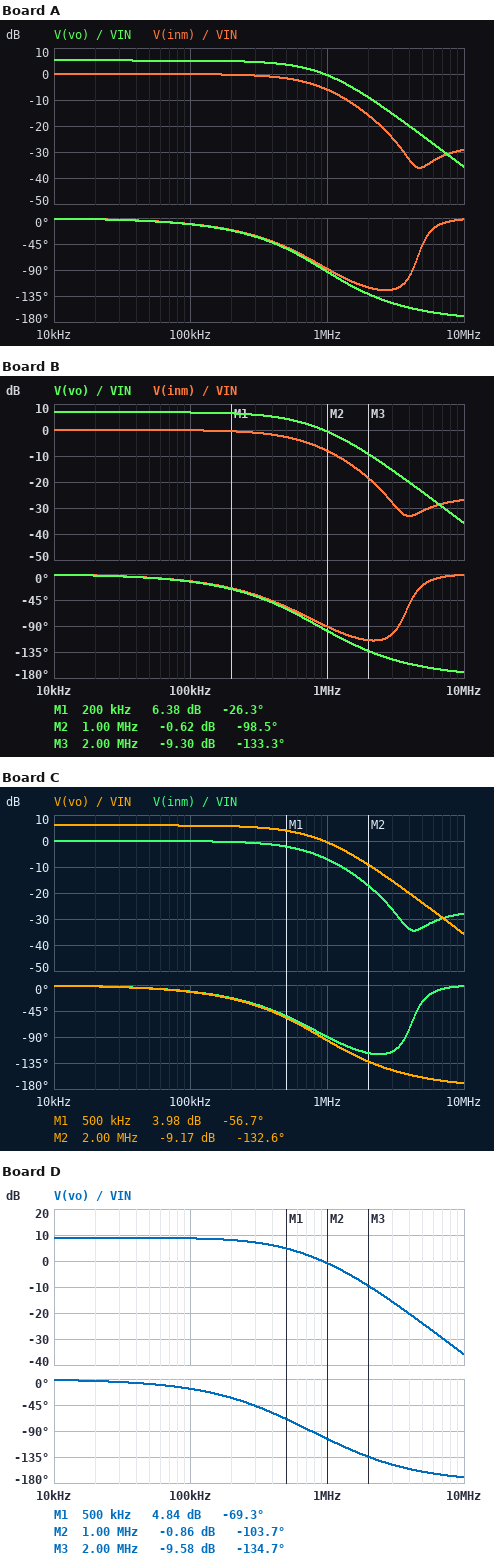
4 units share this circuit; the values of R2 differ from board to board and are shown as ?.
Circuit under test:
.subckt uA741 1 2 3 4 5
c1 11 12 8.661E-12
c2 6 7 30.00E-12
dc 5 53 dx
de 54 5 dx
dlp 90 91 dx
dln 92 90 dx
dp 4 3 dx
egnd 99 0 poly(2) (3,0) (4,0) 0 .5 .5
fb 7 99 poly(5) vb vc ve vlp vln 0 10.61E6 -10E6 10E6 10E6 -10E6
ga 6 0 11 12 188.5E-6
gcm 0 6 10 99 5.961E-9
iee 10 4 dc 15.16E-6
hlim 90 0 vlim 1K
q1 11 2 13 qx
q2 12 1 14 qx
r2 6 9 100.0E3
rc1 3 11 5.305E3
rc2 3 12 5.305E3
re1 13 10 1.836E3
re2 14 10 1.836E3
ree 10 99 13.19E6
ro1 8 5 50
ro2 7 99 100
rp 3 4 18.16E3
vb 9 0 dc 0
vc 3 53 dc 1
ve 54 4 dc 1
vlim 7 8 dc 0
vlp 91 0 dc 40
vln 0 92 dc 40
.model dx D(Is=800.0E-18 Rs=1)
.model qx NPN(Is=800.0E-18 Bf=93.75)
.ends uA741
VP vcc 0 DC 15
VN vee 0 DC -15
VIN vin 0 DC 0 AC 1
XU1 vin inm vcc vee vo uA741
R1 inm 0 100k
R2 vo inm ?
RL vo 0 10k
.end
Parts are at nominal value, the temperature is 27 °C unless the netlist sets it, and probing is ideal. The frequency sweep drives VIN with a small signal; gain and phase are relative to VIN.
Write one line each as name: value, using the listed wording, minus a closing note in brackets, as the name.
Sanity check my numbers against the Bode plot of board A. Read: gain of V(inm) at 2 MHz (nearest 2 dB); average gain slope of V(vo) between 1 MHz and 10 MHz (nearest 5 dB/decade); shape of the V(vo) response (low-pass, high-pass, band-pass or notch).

gain of V(inm) at 2 MHz: -16 dB
average gain slope of V(vo) between 1 MHz and 10 MHz: -35 dB/decade
shape of the V(vo) response: low-pass
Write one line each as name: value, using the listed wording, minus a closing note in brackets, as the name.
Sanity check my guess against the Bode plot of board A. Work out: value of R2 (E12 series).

value of R2: 82 kΩ
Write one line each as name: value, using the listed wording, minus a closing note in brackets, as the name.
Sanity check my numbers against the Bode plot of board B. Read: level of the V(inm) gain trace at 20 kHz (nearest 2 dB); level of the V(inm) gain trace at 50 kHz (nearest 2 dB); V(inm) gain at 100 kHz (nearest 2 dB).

level of the V(inm) gain trace at 20 kHz: 0 dB
level of the V(inm) gain trace at 50 kHz: 0 dB
V(inm) gain at 100 kHz: 0 dB
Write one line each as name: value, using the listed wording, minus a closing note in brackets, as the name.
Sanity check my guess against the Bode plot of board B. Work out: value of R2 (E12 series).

value of R2: 120 kΩ
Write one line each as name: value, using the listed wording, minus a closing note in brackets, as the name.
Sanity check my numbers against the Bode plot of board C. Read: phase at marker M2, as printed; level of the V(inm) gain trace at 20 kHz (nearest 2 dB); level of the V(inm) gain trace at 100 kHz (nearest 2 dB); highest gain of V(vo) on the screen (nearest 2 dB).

phase at marker M2, as printed: -132.6 deg
level of the V(inm) gain trace at 20 kHz: 0 dB
level of the V(inm) gain trace at 100 kHz: 0 dB
highest gain of V(vo) on the screen: 6 dB
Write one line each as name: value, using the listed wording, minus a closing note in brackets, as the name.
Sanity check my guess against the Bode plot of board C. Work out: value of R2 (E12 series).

value of R2: 100 kΩ
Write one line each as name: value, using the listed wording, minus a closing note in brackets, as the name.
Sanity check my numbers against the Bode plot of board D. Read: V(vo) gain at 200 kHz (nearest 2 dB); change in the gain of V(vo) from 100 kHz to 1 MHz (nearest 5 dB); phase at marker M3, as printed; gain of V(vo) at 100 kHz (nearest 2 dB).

V(vo) gain at 200 kHz: 8 dB
change in the gain of V(vo) from 100 kHz to 1 MHz: -10 dB
phase at marker M3, as printed: -134.7 deg
gain of V(vo) at 100 kHz: 8 dB
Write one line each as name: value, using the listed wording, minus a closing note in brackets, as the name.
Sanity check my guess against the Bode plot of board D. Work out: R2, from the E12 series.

R2, from the E12 series: 180 kΩ
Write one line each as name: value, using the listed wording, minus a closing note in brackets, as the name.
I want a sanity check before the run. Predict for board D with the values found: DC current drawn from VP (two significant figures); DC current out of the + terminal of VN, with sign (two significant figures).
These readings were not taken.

DC current drawn from VP: 1.7 mA
DC current out of the + terminal of VN, with sign: -1.7 mA
